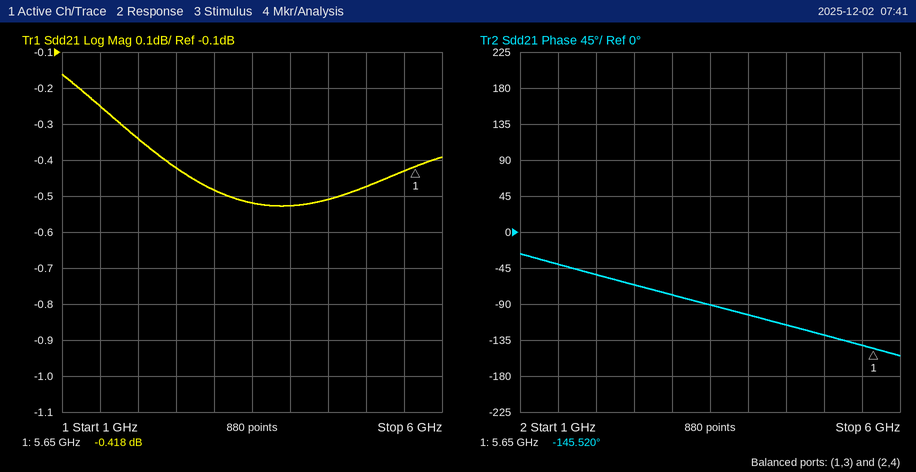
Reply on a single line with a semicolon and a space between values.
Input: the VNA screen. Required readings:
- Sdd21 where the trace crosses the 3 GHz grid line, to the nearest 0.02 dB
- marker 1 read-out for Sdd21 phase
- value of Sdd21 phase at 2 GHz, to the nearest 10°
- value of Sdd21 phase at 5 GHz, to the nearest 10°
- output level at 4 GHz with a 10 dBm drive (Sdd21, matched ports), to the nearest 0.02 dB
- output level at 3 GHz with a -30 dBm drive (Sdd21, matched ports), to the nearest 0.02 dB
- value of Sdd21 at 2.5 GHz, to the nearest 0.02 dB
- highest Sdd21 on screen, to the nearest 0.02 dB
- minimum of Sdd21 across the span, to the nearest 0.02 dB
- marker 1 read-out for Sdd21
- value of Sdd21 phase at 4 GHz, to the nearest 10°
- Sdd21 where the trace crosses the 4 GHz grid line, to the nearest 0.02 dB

-0.48 dB; -145.520°; -50°; -130°; 9.48 dBm; -30.48 dBm; -0.42 dB; -0.16 dB; -0.52 dB; -0.418 dB; -100°; -0.52 dB
